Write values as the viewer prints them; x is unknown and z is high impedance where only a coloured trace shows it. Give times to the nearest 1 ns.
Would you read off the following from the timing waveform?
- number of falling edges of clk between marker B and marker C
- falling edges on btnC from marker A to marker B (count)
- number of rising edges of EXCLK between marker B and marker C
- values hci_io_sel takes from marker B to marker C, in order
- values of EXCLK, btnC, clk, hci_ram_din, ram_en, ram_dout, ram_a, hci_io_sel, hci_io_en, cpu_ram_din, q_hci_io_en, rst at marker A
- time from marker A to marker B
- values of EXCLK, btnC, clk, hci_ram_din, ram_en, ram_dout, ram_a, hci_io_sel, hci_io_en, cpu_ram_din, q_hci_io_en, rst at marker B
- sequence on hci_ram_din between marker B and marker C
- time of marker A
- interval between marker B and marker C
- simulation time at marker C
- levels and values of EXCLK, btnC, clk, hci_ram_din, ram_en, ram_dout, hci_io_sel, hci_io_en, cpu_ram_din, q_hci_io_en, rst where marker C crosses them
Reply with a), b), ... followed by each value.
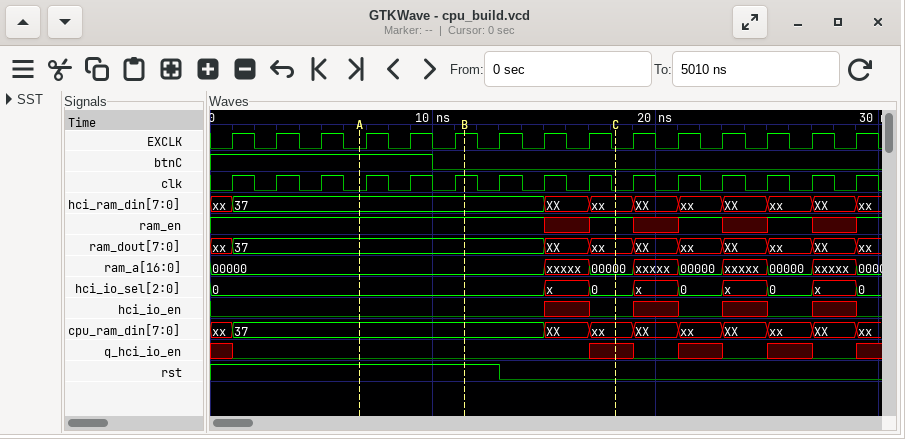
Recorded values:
a) 4
b) 1
c) 3
d) 0, x, 0
e) EXCLK=0, btnC=1, clk=0, hci_ram_din=37, ram_en=1, ram_dout=37, ram_a=00000, hci_io_sel=0, hci_io_en=0, cpu_ram_din=37, q_hci_io_en=0, rst=1
f) 5 ns
g) EXCLK=1, btnC=0, clk=1, hci_ram_din=37, ram_en=1, ram_dout=37, ram_a=00000, hci_io_sel=0, hci_io_en=0, cpu_ram_din=37, q_hci_io_en=0, rst=1
h) 37, XX, xx
i) 7 ns
j) 7 ns
k) 18 ns
l) EXCLK=0, btnC=0, clk=0, hci_ram_din=xx, ram_en=1, ram_dout=xx, hci_io_sel=0, hci_io_en=0, cpu_ram_din=xx, q_hci_io_en=x, rst=0
